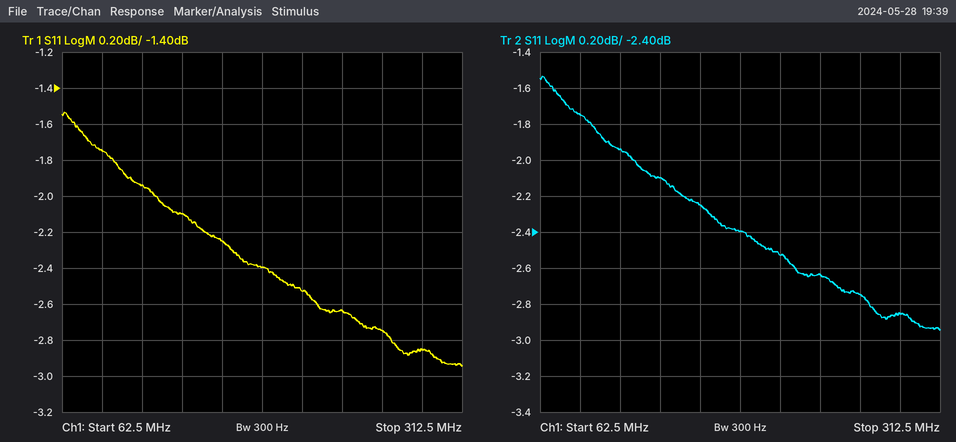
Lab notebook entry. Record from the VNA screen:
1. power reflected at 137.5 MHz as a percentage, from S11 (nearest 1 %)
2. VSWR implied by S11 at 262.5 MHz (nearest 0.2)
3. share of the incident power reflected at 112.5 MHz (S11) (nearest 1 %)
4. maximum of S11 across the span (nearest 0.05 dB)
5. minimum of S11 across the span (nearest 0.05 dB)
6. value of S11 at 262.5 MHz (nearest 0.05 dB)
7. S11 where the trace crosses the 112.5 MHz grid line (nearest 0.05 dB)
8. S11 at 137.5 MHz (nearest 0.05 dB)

62 %
6.4
64 %
-1.55 dB
-2.95 dB
-2.75 dB
-1.95 dB
-2.10 dB
